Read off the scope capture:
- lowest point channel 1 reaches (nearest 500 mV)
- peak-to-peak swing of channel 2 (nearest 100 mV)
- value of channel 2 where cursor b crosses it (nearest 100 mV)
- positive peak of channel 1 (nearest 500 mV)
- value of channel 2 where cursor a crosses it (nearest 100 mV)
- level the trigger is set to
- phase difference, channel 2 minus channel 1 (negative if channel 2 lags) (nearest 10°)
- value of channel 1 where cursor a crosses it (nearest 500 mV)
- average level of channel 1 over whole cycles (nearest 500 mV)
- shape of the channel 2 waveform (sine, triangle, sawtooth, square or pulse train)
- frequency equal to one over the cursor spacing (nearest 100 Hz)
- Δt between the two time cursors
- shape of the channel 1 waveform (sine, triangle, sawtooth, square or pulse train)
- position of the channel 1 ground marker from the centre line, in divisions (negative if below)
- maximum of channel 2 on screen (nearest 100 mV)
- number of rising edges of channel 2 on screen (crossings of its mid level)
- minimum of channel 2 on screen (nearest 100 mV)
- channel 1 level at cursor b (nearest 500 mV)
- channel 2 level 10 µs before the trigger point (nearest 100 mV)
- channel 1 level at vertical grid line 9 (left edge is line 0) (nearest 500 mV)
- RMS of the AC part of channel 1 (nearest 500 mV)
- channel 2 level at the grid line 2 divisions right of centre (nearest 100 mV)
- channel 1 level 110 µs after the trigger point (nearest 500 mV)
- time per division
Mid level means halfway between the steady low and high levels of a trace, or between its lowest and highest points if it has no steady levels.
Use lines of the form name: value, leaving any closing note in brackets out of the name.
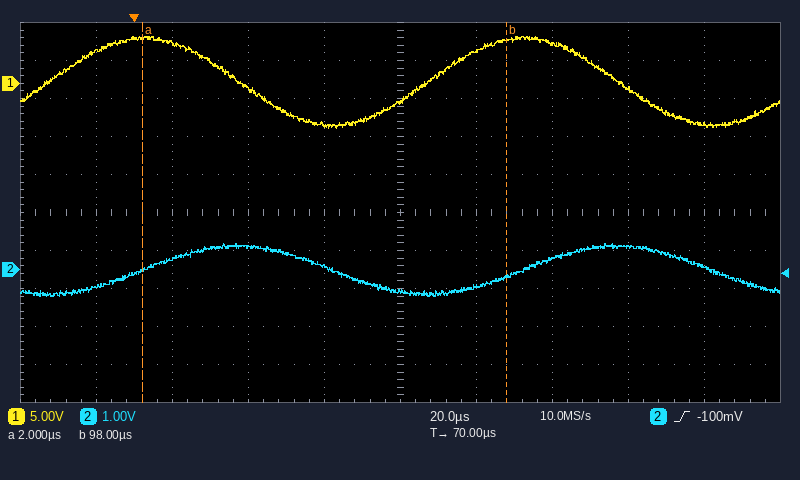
lowest point channel 1 reaches: -6.0 V
peak-to-peak swing of channel 2: 1.4 V
value of channel 2 where cursor b crosses it: -200 mV
positive peak of channel 1: 6.0 V
value of channel 2 where cursor a crosses it: 0.0 V
level the trigger is set to: -100 mV
phase difference, channel 2 minus channel 1 (negative if channel 2 lags): -90°
value of channel 1 where cursor a crosses it: 6.0 V
average level of channel 1 over whole cycles: 0.0 V
shape of the channel 2 waveform: sine
frequency equal to one over the cursor spacing: 10.4 kHz
Δt between the two time cursors: 96 µs
shape of the channel 1 waveform: sine
position of the channel 1 ground marker from the centre line, in divisions: +3.4 div
maximum of channel 2 on screen: 700 mV
number of rising edges of channel 2 on screen: 2
minimum of channel 2 on screen: -700 mV
channel 1 level at cursor b: 5.5 V
channel 2 level 10 µs before the trigger point: -400 mV
channel 1 level at vertical grid line 9 (left edge is line 0): -5.5 V
RMS of the AC part of channel 1: 4.0 V
channel 2 level at the grid line 2 divisions right of centre: 300 mV
channel 1 level 110 µs after the trigger point: 5.0 V
time per division: 20 µs
